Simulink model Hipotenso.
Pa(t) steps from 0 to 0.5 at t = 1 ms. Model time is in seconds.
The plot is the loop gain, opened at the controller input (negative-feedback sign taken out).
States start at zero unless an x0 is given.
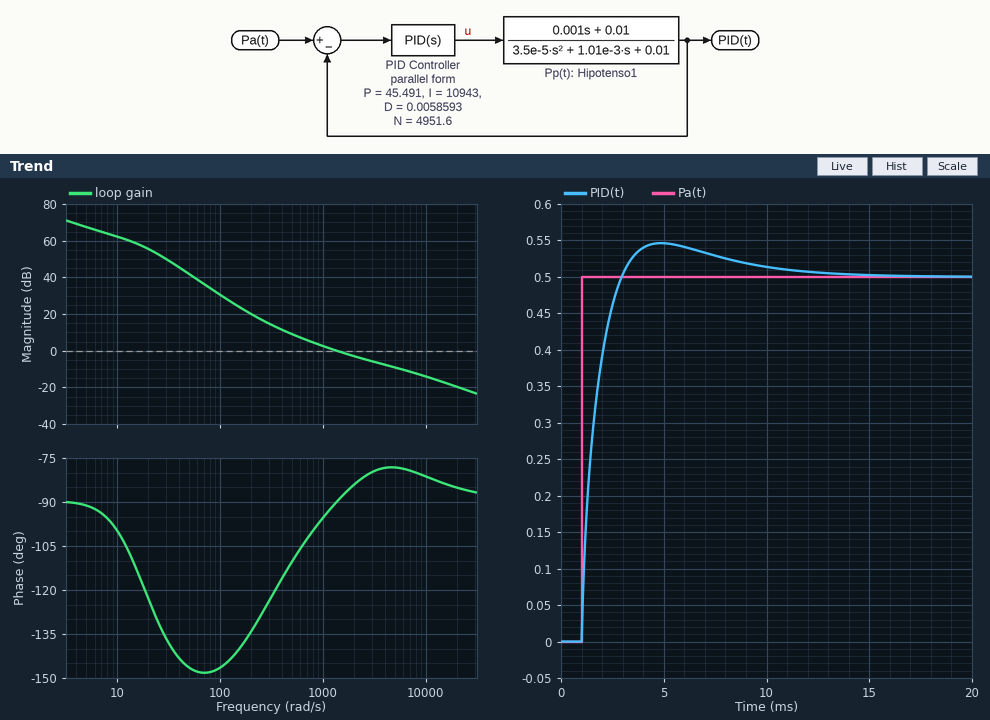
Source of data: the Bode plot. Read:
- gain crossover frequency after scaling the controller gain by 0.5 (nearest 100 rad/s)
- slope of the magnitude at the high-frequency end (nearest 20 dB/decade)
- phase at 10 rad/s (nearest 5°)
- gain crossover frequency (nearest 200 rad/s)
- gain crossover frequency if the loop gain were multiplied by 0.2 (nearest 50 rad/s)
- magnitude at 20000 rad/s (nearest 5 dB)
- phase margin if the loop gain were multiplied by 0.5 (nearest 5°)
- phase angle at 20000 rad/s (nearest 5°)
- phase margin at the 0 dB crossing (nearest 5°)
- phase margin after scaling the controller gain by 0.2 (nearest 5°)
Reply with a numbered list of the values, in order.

1. 700 rad/s
2. -20 dB/decade
3. -100°
4. 1400 rad/s
5. 300 rad/s
6. -20 dB
7. 75°
8. -85°
9. 90°
10. 60°
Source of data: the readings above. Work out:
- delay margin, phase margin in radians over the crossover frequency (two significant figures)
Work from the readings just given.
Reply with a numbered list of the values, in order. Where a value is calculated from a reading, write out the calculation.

1. 90 × π / 180 / 1400 = 0.0011 s
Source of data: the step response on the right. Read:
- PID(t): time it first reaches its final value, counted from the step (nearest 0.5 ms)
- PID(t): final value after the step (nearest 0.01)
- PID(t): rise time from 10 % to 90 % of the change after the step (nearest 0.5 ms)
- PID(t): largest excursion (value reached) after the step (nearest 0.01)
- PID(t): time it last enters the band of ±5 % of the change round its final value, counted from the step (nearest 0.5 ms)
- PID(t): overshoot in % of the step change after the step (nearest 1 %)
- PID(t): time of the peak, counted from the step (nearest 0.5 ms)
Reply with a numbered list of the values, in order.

1. 2.0 ms
2. 0.50
3. 1.5 ms
4. 0.55
5. 7.0 ms
6. 9 %
7. 4.0 ms
